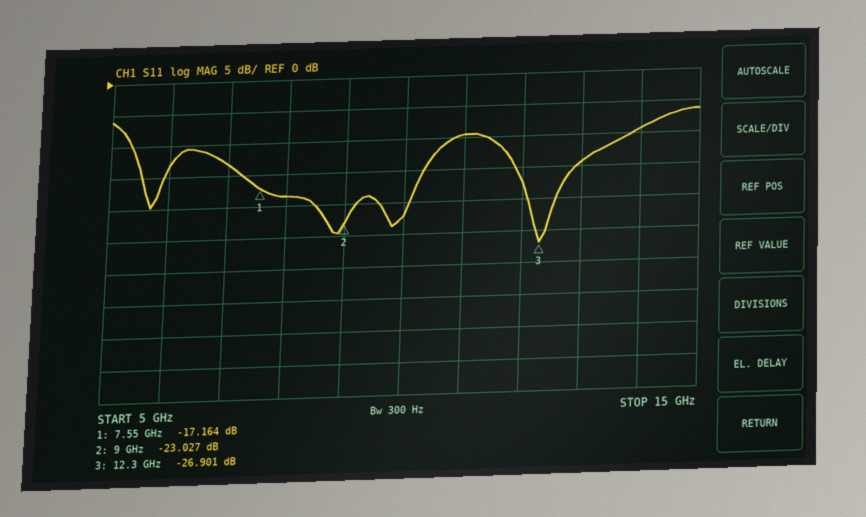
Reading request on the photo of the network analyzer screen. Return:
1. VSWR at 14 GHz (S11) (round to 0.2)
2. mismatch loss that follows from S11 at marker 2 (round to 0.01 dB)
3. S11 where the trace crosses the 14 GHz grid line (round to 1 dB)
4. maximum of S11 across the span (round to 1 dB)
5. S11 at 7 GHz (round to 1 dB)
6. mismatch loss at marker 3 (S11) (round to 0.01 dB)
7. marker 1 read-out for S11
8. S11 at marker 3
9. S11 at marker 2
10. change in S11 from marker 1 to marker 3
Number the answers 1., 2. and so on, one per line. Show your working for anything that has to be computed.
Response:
1. |Γ| = 10^(-9/20) = 0.3548; VSWR = (1 + 0.3548)/(1 − 0.3548) ≈ 2.10, so 2.0 to the nearest 0.2
2. −10 log10(1 − 10^(-23.027/10)) ≈ 0.02 dB
3. -9 dB
4. -6 dB
5. -13 dB
6. −10 log10(1 − 10^(-26.901/10)) ≈ 0.01 dB
7. -17.164 dB
8. -26.901 dB
9. -23.027 dB
10. -26.901 − (-17.164) = -9.737 dB
